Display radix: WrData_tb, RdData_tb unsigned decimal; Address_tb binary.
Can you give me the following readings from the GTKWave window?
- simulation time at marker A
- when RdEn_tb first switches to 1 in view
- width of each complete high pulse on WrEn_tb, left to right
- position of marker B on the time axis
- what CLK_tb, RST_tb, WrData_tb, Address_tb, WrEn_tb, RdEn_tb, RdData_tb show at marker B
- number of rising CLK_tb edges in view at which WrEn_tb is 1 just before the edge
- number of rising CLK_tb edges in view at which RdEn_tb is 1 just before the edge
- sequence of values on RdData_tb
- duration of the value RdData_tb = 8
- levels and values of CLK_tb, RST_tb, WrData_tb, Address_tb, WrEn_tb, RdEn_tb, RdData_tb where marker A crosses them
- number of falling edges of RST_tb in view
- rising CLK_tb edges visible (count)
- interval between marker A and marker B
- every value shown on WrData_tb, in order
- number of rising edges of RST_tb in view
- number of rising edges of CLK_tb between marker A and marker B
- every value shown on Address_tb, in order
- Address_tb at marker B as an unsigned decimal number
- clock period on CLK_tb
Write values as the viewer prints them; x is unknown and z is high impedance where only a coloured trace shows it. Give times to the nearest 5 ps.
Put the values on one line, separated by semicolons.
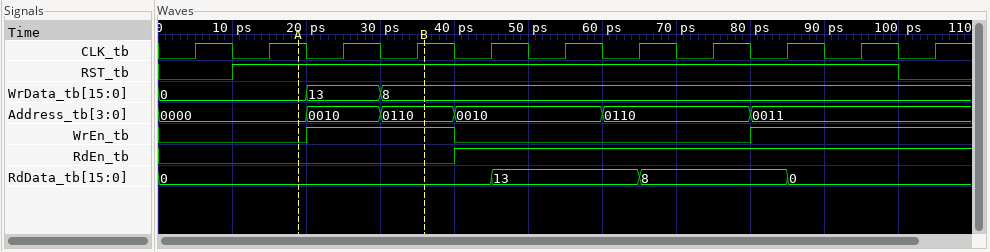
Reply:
20 ps; 40 ps; 20 ps; 35 ps; CLK_tb=1, RST_tb=1, WrData_tb=8, Address_tb=0110, WrEn_tb=1, RdEn_tb=0, RdData_tb=0; 5; 7; 0, 13, 8, 0; 20 ps; CLK_tb=1, RST_tb=1, WrData_tb=0, Address_tb=0000, WrEn_tb=0, RdEn_tb=0, RdData_tb=0; 1; 11; 15 ps; 0, 13, 8; 1; 2; 0000, 0010, 0110, 0010, 0110, 0011; 6; 10 ps
